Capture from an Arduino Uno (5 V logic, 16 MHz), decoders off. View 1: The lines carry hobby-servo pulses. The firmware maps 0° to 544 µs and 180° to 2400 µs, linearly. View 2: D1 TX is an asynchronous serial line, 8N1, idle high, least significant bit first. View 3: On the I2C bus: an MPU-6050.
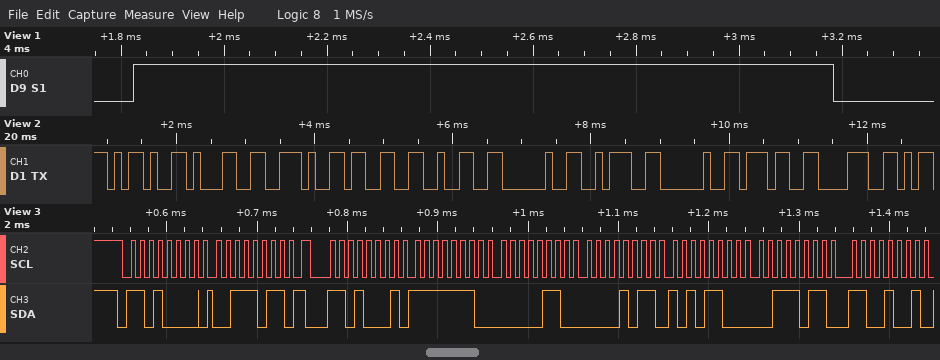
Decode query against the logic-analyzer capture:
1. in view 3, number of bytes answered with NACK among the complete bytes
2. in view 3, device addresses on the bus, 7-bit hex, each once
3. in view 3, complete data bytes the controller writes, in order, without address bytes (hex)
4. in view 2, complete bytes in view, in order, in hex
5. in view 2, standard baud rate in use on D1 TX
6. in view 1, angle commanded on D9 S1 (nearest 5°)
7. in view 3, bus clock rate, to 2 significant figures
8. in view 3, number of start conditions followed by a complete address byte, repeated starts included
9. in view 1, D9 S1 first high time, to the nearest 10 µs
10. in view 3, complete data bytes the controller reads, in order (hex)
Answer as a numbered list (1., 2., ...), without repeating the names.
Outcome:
1. 0
2. 0x68
3. 3B
4. 2D 31 2E 33 32 20 3A 20 37 38
5. 9600 baud
6. 80°
7. 100 kHz
8. 2
9. 1360 µs
10. FE 06 0B AC 3B C9
